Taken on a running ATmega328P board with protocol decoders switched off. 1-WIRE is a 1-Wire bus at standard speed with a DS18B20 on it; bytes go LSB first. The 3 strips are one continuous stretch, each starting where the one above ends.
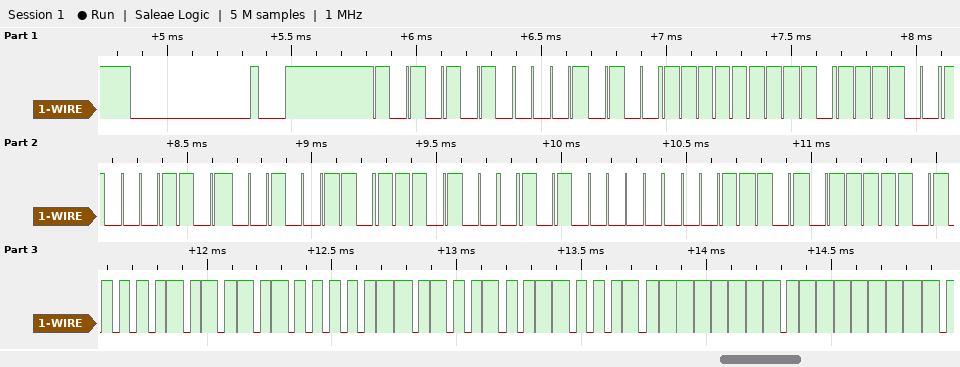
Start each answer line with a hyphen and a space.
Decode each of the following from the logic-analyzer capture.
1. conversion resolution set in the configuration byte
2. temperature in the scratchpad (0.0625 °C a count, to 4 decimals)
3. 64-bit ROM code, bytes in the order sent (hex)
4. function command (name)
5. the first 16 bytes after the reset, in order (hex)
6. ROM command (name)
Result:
- 12 bits
- 85.0000 °C
- 28 FF 3D B1 64 17 05 B8
- Read Scratchpad
- 55 28 FF 3D B1 64 17 05 B8 BE 50 05 4B 46 7F FF
- Match ROM
